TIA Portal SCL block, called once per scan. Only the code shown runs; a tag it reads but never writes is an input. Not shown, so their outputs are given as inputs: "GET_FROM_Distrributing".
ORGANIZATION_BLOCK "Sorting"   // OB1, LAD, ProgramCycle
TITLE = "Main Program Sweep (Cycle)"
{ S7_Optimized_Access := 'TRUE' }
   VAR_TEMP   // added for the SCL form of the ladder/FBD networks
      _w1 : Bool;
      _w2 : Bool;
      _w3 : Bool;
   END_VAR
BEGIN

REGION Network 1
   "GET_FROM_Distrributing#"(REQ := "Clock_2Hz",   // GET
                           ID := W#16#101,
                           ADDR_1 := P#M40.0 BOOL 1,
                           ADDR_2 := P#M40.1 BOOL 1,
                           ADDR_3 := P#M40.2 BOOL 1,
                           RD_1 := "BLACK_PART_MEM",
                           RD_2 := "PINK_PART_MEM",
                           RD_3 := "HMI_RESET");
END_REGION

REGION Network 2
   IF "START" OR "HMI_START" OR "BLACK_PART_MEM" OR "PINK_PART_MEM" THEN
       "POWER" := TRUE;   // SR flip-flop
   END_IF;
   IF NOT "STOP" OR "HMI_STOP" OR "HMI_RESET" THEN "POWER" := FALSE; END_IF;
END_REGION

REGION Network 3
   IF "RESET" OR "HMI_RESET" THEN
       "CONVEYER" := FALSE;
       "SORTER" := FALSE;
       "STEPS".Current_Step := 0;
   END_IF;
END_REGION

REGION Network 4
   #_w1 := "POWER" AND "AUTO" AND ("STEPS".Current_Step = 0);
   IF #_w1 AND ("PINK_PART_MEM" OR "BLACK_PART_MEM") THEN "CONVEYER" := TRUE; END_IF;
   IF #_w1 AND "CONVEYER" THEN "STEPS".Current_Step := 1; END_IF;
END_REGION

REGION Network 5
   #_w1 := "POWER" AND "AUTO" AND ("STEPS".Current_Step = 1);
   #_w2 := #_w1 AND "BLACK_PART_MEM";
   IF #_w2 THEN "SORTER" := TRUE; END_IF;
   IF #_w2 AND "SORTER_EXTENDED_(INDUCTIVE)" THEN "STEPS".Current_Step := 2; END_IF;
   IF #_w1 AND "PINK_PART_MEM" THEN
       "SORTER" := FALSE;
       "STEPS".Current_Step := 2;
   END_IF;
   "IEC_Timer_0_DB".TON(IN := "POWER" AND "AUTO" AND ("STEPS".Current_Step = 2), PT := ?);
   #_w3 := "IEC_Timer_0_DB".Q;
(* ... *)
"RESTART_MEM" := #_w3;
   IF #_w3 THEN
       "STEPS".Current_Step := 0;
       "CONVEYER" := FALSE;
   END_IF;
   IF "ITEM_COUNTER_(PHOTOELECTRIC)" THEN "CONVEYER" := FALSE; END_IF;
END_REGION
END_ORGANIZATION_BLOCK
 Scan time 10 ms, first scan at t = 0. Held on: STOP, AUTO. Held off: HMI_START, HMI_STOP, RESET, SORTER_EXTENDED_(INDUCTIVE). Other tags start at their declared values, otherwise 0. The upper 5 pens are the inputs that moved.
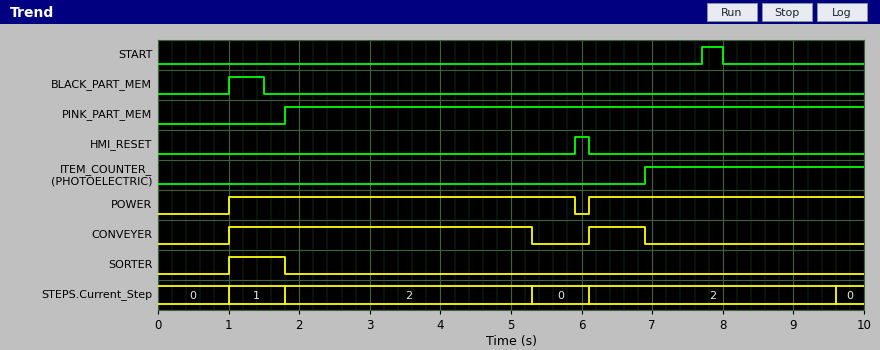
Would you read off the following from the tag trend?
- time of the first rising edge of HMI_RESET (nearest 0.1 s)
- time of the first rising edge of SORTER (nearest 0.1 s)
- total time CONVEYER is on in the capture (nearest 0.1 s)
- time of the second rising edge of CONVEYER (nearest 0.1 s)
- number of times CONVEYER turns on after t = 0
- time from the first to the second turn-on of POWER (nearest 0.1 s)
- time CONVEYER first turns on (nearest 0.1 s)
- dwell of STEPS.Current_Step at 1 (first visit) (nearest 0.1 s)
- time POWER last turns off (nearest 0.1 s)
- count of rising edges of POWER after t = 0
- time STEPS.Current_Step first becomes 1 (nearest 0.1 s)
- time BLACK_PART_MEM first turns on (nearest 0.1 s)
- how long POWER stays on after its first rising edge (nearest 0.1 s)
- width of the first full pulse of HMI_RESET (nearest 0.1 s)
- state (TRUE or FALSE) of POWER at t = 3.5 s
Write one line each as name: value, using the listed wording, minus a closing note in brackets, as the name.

time of the first rising edge of HMI_RESET: 5.9 s
time of the first rising edge of SORTER: 1.0 s
total time CONVEYER is on in the capture: 5.1 s
time of the second rising edge of CONVEYER: 6.1 s
number of times CONVEYER turns on after t = 0: 2
time from the first to the second turn-on of POWER: 5.1 s
time CONVEYER first turns on: 1.0 s
dwell of STEPS.Current_Step at 1 (first visit): 0.8 s
time POWER last turns off: 5.9 s
count of rising edges of POWER after t = 0: 2
time STEPS.Current_Step first becomes 1: 1.0 s
time BLACK_PART_MEM first turns on: 1.0 s
how long POWER stays on after its first rising edge: 4.9 s
width of the first full pulse of HMI_RESET: 0.2 s
state (TRUE or FALSE) of POWER at t = 3.5 s: TRUE
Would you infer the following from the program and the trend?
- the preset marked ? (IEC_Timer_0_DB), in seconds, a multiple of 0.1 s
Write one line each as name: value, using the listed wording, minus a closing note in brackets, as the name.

the preset marked ? (IEC_Timer_0_DB), in seconds, a multiple of 0.1 s: 3.5 s
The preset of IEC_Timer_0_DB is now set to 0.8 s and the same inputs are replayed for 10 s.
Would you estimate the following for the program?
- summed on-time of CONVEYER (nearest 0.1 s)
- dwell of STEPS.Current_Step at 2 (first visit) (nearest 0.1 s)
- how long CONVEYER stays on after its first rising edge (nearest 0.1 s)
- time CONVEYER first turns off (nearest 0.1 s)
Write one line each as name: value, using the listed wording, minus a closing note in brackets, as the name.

summed on-time of CONVEYER: 2.4 s
dwell of STEPS.Current_Step at 2 (first visit): 0.8 s
how long CONVEYER stays on after its first rising edge: 1.6 s
time CONVEYER first turns off: 2.6 s
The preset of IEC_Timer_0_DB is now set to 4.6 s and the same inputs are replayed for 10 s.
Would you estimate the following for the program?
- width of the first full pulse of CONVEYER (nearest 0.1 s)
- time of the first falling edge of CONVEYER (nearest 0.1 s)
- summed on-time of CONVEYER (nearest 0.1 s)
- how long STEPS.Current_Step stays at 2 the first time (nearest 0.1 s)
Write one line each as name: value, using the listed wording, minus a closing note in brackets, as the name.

width of the first full pulse of CONVEYER: 4.9 s
time of the first falling edge of CONVEYER: 5.9 s
summed on-time of CONVEYER: 5.7 s
how long STEPS.Current_Step stays at 2 the first time: 4.1 s
